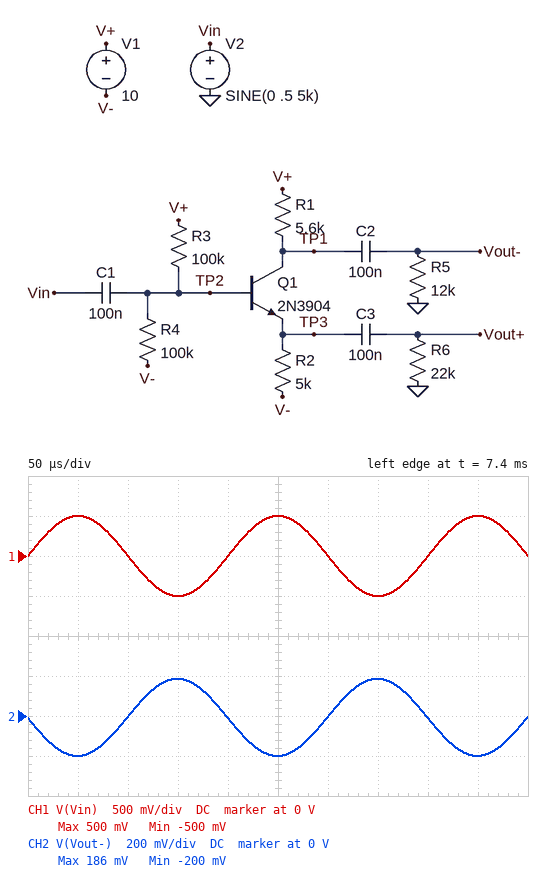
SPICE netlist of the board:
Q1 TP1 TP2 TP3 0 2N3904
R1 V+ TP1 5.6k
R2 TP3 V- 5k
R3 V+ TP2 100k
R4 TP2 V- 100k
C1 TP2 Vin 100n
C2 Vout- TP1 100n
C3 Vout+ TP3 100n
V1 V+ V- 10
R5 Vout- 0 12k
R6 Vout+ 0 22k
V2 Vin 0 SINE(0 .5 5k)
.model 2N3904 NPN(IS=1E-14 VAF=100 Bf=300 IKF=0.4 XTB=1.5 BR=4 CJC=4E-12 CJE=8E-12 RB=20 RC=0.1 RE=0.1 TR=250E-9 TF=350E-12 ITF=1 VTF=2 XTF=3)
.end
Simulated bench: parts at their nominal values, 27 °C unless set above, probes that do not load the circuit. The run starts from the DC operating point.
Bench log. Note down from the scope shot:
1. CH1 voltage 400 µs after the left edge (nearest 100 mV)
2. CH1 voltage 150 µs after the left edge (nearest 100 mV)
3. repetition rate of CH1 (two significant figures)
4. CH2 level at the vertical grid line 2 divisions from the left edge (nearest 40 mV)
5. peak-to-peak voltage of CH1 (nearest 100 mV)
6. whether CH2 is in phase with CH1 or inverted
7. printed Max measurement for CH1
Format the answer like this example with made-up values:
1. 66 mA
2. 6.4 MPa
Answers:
1. 0 V
2. -500 mV
3. 5.0 kHz
4. 0 V
5. 1.0 V
6. inverted
7. 500 mV
